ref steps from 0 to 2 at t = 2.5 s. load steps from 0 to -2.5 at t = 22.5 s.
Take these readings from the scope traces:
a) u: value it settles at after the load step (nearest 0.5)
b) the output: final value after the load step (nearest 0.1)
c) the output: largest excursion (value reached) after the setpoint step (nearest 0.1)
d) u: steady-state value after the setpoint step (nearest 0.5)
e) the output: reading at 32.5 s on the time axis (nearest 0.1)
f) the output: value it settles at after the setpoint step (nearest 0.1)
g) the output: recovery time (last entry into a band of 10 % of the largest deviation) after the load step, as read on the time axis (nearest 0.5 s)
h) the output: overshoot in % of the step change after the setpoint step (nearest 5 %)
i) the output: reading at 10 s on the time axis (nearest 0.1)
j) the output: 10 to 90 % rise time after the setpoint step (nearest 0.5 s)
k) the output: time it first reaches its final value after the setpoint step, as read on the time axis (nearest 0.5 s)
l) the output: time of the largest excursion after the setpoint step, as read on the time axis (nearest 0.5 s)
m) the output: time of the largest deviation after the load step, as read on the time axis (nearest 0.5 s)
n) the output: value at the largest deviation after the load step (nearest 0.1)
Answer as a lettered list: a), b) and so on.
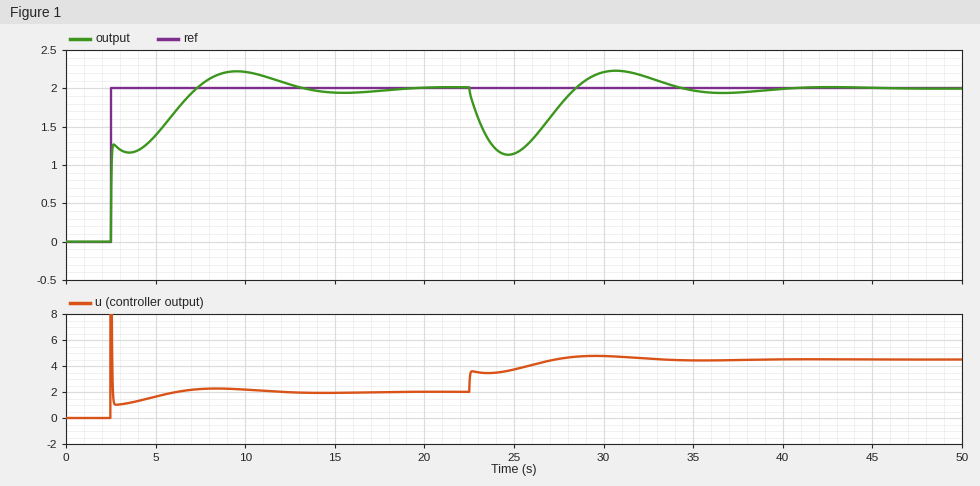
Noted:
a) 4.5
b) 2.0
c) 2.2
d) 2.0
e) 2.1
f) 2.0
g) 33.0 s
h) 10 %
i) 2.2
j) 4.0 s
k) 7.5 s
l) 9.5 s
m) 24.5 s
n) 1.1
